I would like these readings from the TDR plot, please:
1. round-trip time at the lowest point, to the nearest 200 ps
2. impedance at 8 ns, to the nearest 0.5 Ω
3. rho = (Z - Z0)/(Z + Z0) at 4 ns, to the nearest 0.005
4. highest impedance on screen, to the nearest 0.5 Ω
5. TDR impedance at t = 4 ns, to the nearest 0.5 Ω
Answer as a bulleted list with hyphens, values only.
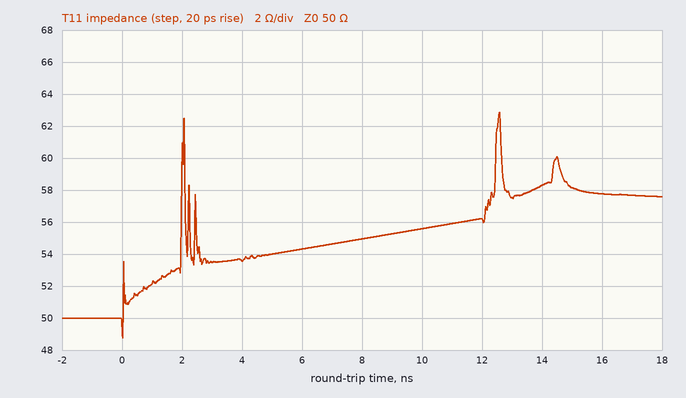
- 0.0 ns
- 55.0 Ω
- +0.035
- 63.0 Ω
- 53.5 Ω
